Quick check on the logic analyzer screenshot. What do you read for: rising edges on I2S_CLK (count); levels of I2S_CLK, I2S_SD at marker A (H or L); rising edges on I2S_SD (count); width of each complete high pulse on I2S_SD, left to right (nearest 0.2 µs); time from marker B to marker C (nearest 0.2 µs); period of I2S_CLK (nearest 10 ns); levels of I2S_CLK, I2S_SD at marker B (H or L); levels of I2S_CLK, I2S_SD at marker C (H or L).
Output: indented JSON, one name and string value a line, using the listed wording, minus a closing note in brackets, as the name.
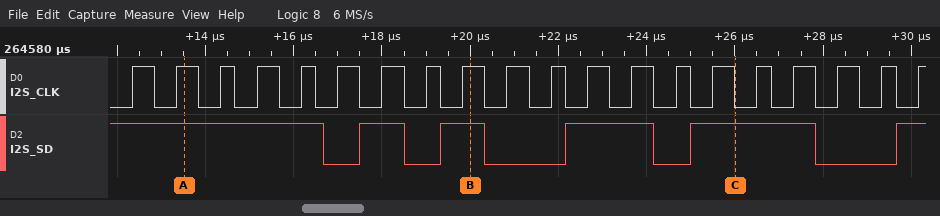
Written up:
{
  "rising edges on I2S_CLK": "20",
  "levels of I2S_CLK, I2S_SD at marker A": "I2S_CLK=H, I2S_SD=H",
  "rising edges on I2S_SD": "5",
  "width of each complete high pulse on I2S_SD, left to right": "1 µs, 1 µs, 2 µs, 2.8 µs",
  "time from marker B to marker C": "6 µs",
  "period of I2S_CLK": "940 ns",
  "levels of I2S_CLK, I2S_SD at marker B": "I2S_CLK=H, I2S_SD=H",
  "levels of I2S_CLK, I2S_SD at marker C": "I2S_CLK=L, I2S_SD=H"
}
